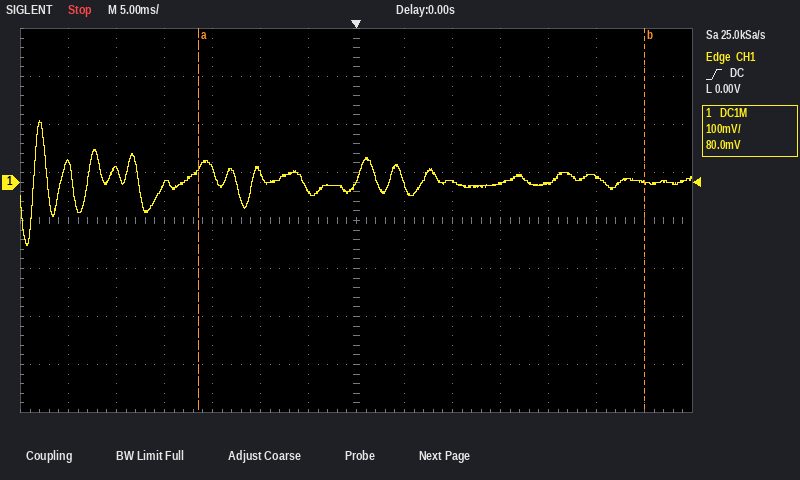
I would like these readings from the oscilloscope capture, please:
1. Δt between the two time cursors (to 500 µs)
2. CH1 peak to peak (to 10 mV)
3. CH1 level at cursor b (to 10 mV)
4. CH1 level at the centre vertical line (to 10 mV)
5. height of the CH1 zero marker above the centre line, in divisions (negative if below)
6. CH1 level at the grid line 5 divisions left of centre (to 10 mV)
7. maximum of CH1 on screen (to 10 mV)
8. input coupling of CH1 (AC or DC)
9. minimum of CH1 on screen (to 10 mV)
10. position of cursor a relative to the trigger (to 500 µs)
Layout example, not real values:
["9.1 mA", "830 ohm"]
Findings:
["46.5 ms", "260 mV", "0 mV", "0 mV", "+0.8 div", "30 mV", "130 mV", "DC", "-130 mV", "-16.5 ms"]
